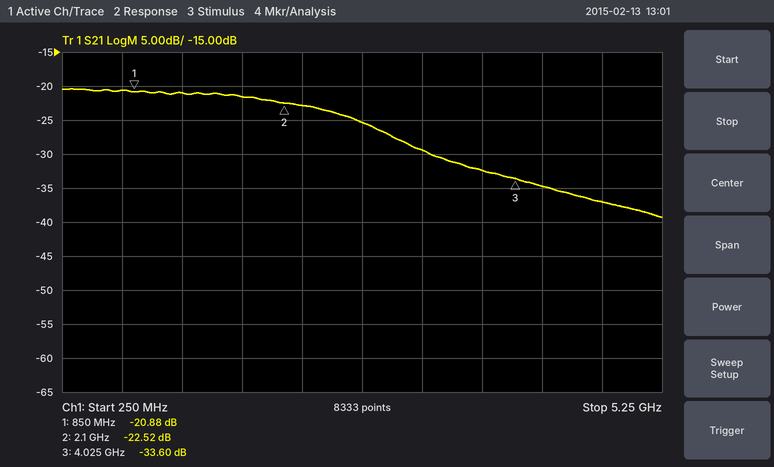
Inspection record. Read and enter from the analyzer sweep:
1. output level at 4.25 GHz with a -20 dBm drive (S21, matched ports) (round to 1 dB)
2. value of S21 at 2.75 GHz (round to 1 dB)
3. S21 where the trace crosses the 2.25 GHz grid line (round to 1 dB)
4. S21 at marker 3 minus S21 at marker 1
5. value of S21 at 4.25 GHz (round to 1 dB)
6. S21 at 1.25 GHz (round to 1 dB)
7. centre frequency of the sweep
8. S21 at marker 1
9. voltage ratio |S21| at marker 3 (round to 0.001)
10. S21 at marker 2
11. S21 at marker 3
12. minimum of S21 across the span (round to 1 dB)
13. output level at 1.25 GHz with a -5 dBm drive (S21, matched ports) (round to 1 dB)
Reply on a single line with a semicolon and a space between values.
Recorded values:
-55 dBm; -25 dB; -23 dB; -12.72 dB; -35 dB; -21 dB; 2.75 GHz; -20.88 dB; 0.021; -22.52 dB; -33.60 dB; -39 dB; -26 dBm
